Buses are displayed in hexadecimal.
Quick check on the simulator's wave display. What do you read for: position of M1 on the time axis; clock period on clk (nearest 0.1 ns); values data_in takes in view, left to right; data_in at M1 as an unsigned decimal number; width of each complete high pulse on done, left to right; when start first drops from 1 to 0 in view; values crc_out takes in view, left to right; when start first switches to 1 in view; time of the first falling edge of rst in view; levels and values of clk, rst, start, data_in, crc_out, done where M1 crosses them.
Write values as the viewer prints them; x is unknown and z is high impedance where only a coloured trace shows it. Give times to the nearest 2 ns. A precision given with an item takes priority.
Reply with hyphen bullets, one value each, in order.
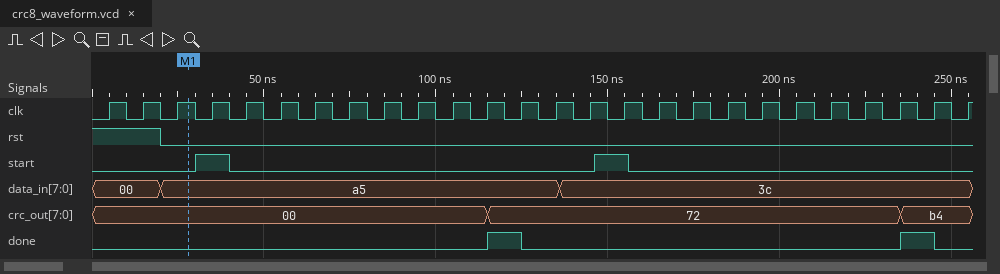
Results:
- 28 ns
- 10 ns
- 00, a5, 3c
- 165
- 10 ns, 10 ns
- 40 ns
- 00, 72, b4
- 30 ns
- 20 ns
- clk=1, rst=0, start=0, data_in=a5, crc_out=00, done=0
